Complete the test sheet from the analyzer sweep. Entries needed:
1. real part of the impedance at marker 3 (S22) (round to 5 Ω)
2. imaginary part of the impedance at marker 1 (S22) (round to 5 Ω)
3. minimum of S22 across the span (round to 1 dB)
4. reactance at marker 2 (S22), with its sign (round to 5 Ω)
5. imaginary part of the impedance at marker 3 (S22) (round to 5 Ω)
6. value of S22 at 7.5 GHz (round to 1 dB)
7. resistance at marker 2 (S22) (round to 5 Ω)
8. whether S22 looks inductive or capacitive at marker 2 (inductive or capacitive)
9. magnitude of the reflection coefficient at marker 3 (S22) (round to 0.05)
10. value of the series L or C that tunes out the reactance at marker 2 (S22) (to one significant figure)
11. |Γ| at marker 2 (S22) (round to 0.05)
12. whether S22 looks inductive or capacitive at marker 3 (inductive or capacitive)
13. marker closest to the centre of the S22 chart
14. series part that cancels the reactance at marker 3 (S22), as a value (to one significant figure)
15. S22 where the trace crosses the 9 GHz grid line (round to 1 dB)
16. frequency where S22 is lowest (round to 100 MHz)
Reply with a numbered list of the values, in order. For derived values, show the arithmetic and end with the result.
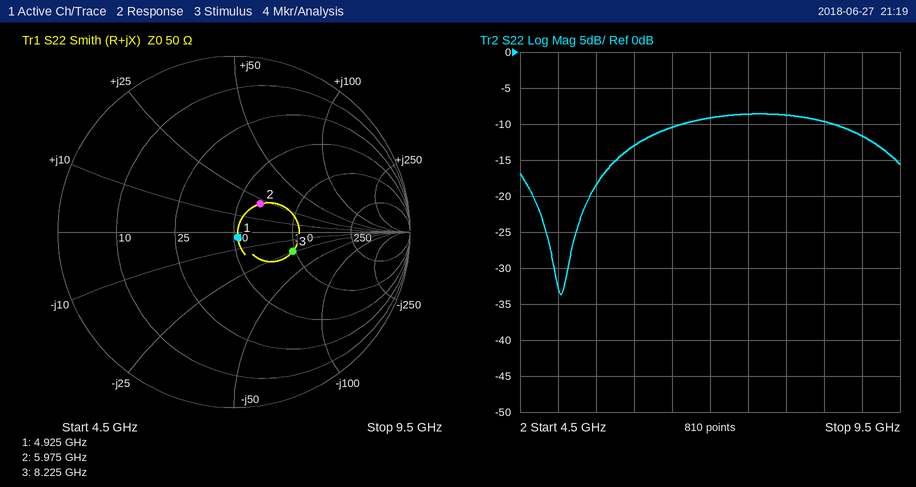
1. 95 Ω
2. -5 Ω
3. -34 dB
4. +20 Ω
5. -25 Ω
6. -9 dB
7. 65 Ω
8. inductive
9. 0.35
10. C = 1/(2π × 5.975 GHz × 20 Ω) ≈ 1 pF
11. 0.20
12. capacitive
13. marker 1
14. L = 25 Ω/(2π × 8.225 GHz) ≈ 484 pH, so 500 pH to one significant figure
15. -12 dB
16. 5.0 GHz
